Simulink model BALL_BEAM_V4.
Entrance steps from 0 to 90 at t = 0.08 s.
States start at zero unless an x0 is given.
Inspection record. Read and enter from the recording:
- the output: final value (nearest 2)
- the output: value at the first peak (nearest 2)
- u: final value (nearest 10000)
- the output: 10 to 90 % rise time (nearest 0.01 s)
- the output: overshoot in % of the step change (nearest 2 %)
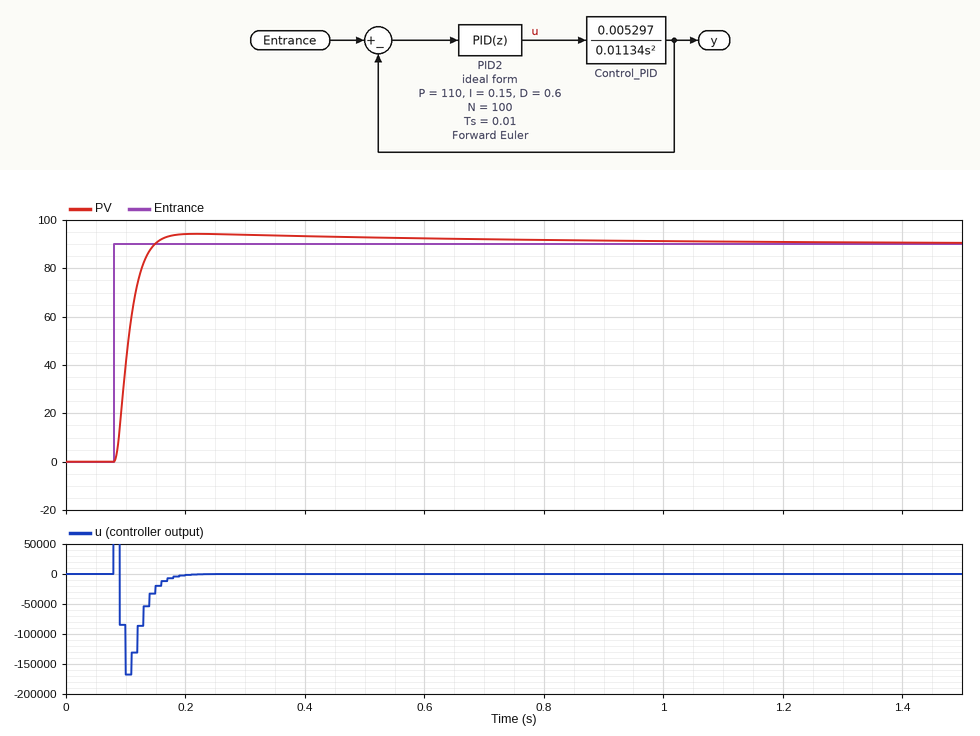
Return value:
90
94
0
0.04 s
4 %
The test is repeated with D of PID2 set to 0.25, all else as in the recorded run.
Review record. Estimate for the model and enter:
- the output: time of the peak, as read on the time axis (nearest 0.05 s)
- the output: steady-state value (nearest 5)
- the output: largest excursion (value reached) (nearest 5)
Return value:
0.35 s
90
105
